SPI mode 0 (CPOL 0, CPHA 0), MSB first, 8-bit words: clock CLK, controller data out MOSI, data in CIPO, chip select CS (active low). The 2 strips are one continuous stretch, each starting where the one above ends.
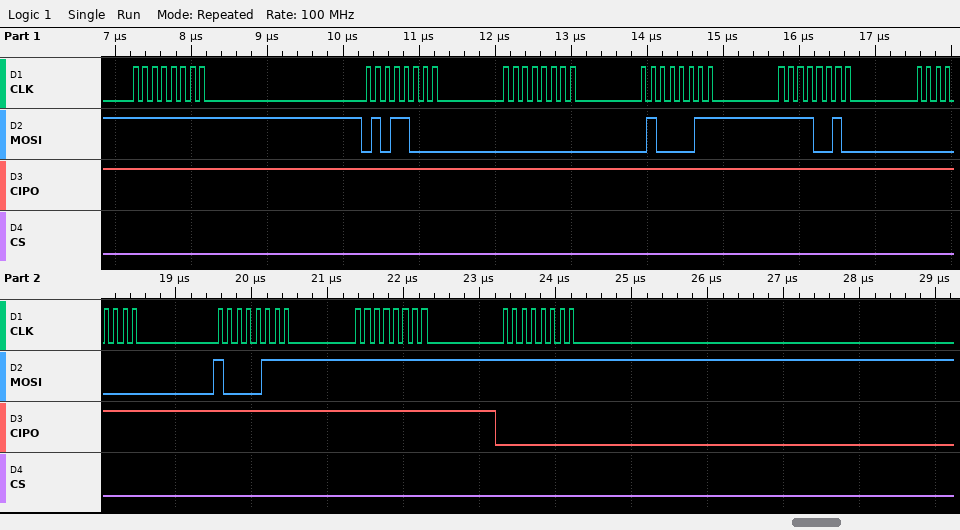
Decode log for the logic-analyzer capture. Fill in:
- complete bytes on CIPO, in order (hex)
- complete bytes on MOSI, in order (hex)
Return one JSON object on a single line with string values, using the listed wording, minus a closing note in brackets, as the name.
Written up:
{"complete bytes on CIPO, in order": "FF FF FF FF FF FF FF FF 00", "complete bytes on MOSI, in order": "FF 58 00 43 F2 00 87 FF FF"}
